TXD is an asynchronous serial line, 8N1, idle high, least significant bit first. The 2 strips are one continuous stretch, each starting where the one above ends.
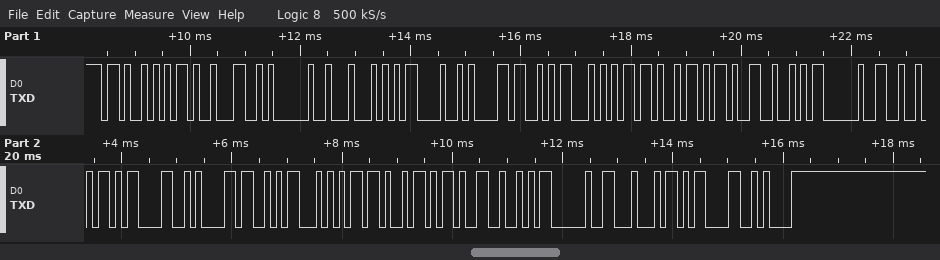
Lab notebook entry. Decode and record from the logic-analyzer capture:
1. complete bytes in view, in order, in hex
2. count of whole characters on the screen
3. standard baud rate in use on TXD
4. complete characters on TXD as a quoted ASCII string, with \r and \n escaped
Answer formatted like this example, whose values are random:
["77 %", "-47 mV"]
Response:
["4B 2D 4C 20 44 0D 0A 53 54 4B 2D 52 20 52 0D 0A 53 54 4B 2D 52 20 44 0D 0A", "25", "9600 baud", "\"K-L D\\r\\nSTK-R R\\r\\nSTK-R D\\r\\n\""]
